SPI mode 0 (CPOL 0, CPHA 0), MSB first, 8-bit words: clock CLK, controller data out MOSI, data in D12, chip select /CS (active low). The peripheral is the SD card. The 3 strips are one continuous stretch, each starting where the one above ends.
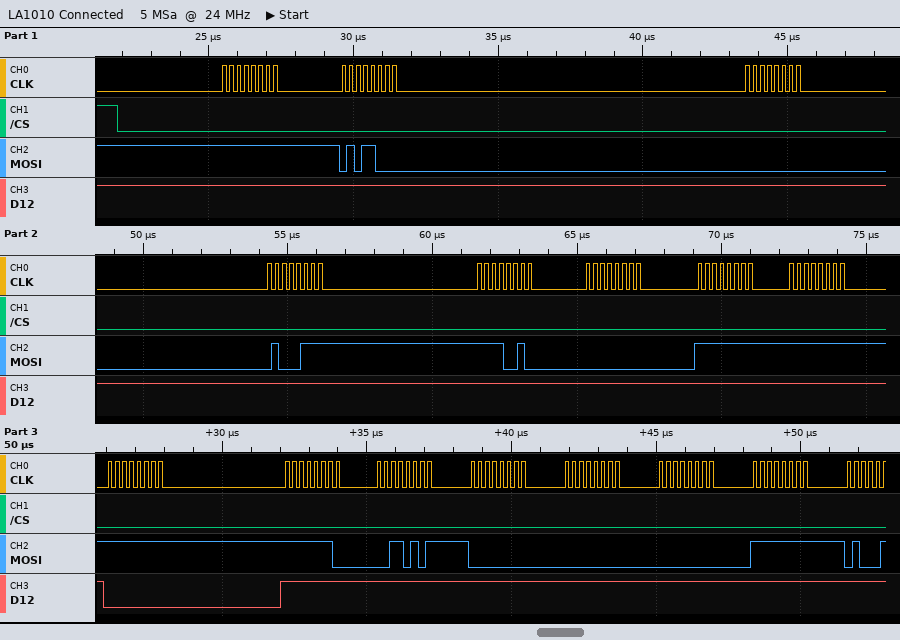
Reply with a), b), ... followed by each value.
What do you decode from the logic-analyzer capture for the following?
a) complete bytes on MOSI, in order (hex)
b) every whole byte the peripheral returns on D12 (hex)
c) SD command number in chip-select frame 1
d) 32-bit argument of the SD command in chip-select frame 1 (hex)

a) FF 58 00 47 F2 00 FF FF FF FE 35 00 00 00 FF
b) FF FF FF FF FF FF FF FF 00 FF FF FF FF FF FF
c) CMD24
d) 0x0047F200
